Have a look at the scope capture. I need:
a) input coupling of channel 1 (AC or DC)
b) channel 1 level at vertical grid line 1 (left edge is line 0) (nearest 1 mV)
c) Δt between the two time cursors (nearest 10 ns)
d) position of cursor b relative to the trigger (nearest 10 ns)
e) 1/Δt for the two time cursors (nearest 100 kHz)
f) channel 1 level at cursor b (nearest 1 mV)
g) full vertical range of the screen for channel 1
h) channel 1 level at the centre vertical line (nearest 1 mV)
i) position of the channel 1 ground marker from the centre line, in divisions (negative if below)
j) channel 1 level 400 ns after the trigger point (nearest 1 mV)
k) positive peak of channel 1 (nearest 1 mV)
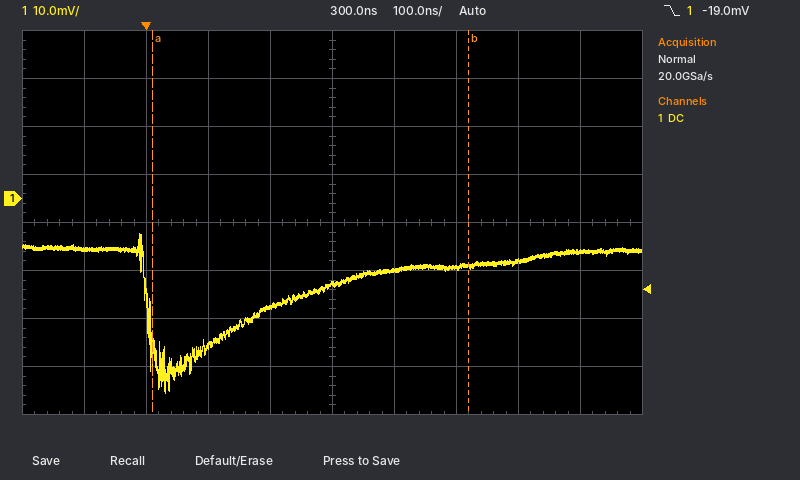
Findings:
DC
-11 mV
510 ns
+520 ns
2.0 MHz
-14 mV
80 mV
-18 mV
+0.5 div
-15 mV
-7 mV
